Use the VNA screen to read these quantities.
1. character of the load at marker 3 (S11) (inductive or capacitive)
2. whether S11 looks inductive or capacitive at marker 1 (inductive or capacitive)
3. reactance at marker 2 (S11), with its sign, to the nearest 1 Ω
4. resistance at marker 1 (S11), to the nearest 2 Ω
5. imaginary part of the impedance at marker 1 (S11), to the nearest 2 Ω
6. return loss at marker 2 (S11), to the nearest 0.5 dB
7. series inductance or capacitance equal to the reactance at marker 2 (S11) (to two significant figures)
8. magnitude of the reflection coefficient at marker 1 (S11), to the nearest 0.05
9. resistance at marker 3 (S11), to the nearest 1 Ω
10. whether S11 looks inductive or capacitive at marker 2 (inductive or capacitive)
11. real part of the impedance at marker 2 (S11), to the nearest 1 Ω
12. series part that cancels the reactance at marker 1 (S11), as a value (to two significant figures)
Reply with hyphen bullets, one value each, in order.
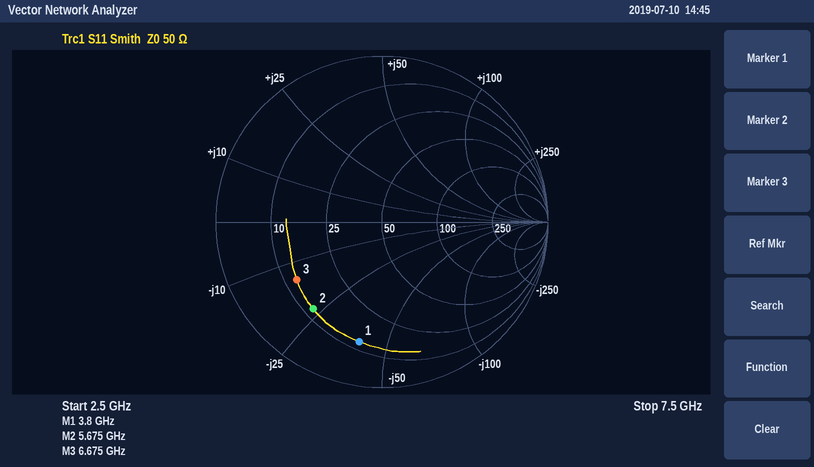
- capacitive
- capacitive
- -23 Ω
- 12 Ω
- -40 Ω
- 3.5 dB
- 1.2 pF
- 0.75
- 13 Ω
- capacitive
- 12 Ω
- 1.7 nH
